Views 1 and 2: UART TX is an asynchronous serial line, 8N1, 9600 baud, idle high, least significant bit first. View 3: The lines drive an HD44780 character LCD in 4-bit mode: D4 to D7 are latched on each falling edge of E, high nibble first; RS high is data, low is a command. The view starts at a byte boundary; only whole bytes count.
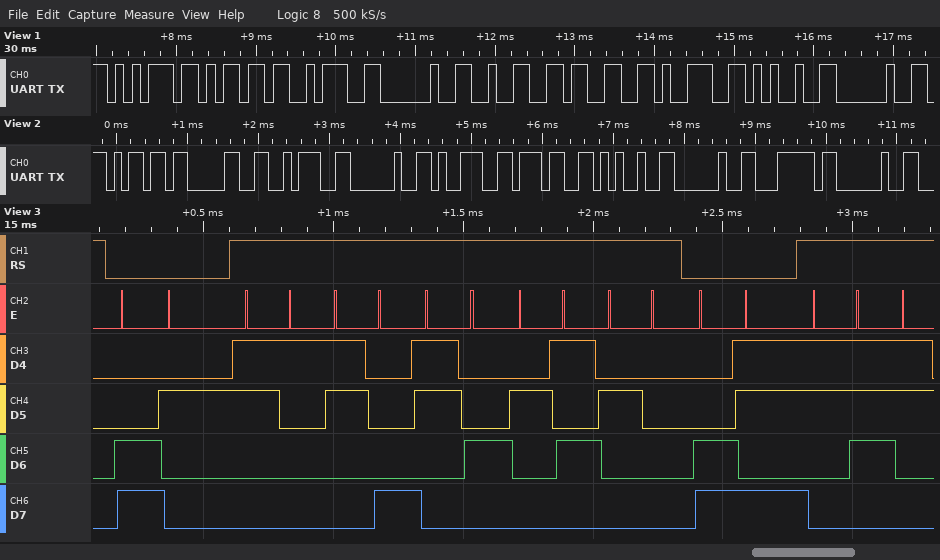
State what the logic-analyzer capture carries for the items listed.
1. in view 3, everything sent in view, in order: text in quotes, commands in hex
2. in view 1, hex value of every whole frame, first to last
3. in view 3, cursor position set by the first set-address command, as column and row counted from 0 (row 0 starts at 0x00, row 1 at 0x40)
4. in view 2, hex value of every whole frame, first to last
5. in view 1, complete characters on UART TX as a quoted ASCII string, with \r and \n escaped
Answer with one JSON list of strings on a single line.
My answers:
["0xC2 \"184% \" 0xCB \"7\"", "75 6D 3A 20 32 33 39 25 20", "column 2, row 1", "6D 30 3A 20 39 37 25 20 7C 20", "\"um: 239% \""]
